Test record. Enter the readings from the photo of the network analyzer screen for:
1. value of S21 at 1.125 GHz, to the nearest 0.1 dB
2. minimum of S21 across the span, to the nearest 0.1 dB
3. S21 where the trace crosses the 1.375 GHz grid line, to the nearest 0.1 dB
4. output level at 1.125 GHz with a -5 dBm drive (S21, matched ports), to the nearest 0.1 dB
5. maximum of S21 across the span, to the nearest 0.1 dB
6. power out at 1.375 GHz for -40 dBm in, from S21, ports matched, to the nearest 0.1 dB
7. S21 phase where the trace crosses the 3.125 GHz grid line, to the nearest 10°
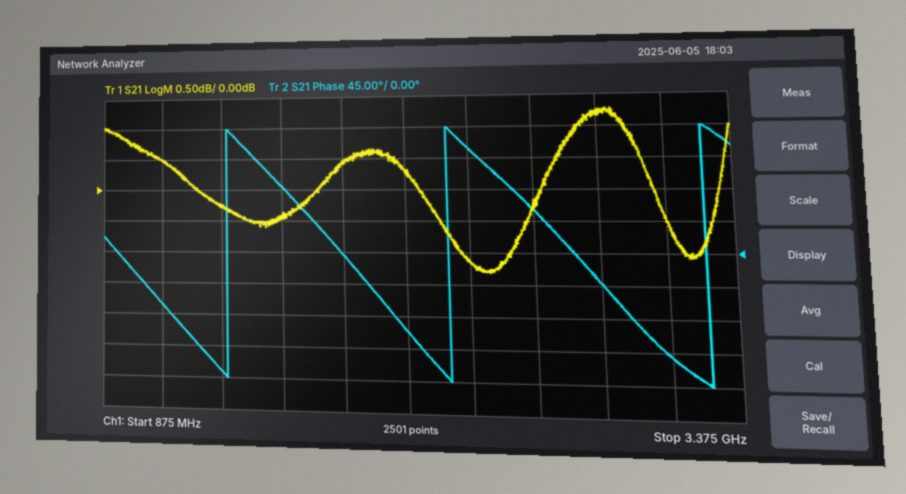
0.5 dB
-1.3 dB
-0.3 dB
-4.5 dBm
1.3 dB
-40.3 dBm
-140°
